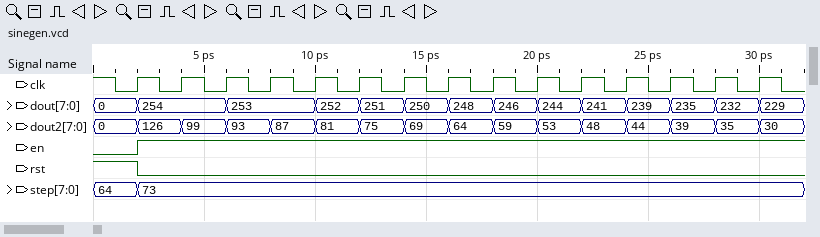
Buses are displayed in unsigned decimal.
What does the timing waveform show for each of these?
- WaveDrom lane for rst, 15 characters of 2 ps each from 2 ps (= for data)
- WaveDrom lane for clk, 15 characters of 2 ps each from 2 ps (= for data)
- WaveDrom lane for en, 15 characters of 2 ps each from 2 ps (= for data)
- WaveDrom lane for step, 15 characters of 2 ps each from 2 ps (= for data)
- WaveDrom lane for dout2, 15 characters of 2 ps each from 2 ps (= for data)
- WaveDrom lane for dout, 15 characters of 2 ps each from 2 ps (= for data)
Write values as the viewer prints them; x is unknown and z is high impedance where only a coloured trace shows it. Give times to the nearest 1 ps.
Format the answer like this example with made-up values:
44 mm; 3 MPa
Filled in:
{name: 'rst', wave: '0..............'}; {name: 'clk', wave: 'p..............'}; {name: 'en', wave: '1..............'}; {name: 'step', wave: '=..............', data: '73'}; {name: 'dout2', wave: '===============', data: '126 99 93 87 81 75 69 64 59 53 48 44 39 35 30'}; {name: 'dout', wave: '=.=.===========', data: '254 253 252 251 250 248 246 244 241 239 235 232 229'}
